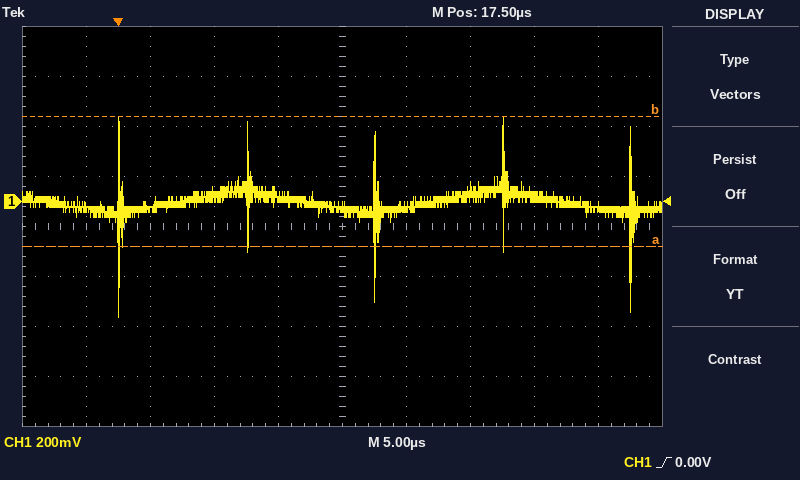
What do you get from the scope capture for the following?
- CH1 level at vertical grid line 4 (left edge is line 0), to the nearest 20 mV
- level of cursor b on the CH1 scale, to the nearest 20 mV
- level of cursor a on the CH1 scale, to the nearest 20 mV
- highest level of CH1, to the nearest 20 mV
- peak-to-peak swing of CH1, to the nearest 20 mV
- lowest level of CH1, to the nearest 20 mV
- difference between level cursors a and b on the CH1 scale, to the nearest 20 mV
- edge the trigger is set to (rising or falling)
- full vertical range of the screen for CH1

20 mV
340 mV
-180 mV
340 mV
800 mV
-460 mV
520 mV
rising
1.6 V
